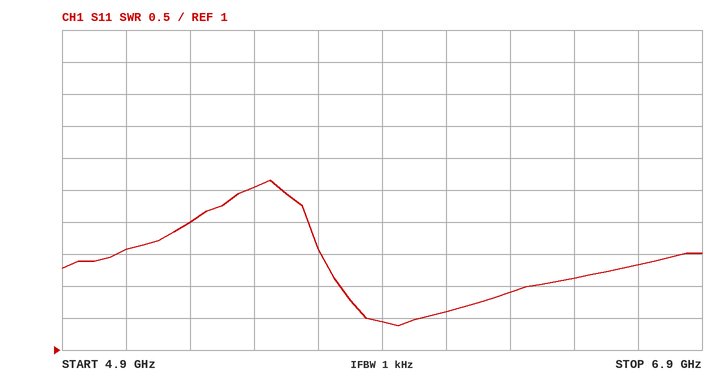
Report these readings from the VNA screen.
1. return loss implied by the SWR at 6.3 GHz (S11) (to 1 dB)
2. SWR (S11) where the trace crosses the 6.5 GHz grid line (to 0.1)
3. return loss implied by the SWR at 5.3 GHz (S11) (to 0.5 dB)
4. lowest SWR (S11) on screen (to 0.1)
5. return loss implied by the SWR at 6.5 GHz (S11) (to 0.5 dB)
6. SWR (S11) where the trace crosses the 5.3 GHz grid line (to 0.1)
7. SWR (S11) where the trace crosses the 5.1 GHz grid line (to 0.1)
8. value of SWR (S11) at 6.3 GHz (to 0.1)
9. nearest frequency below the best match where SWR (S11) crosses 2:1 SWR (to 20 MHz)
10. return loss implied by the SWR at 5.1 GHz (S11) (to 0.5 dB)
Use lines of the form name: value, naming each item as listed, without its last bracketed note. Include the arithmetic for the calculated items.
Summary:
return loss implied by the SWR at 6.3 GHz (S11): −20 log10((1.9 − 1)/(1.9 + 1)) ≈ 10 dB
SWR (S11) where the trace crosses the 6.5 GHz grid line: 2.1
return loss implied by the SWR at 5.3 GHz (S11): −20 log10((3 − 1)/(3 + 1)) ≈ 6.0 dB
lowest SWR (S11) on screen: 1.4
return loss implied by the SWR at 6.5 GHz (S11): −20 log10((2.1 − 1)/(2.1 + 1)) ≈ 9.0 dB
SWR (S11) where the trace crosses the 5.3 GHz grid line: 3.0
SWR (S11) where the trace crosses the 5.1 GHz grid line: 2.6
value of SWR (S11) at 6.3 GHz: 1.9
nearest frequency below the best match where SWR (S11) crosses 2:1 SWR: 5.76 GHz
return loss implied by the SWR at 5.1 GHz (S11): −20 log10((2.6 − 1)/(2.6 + 1)) ≈ 7.0 dB
